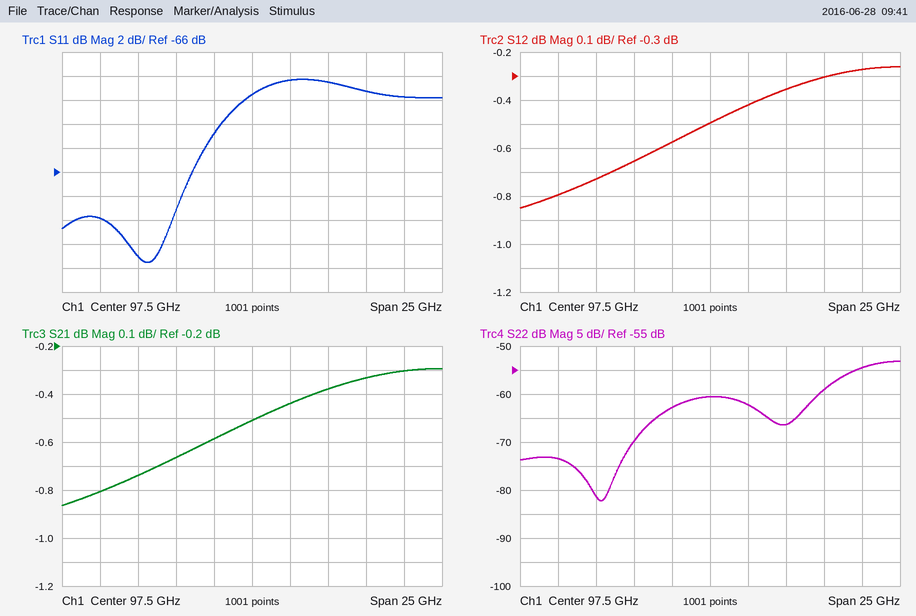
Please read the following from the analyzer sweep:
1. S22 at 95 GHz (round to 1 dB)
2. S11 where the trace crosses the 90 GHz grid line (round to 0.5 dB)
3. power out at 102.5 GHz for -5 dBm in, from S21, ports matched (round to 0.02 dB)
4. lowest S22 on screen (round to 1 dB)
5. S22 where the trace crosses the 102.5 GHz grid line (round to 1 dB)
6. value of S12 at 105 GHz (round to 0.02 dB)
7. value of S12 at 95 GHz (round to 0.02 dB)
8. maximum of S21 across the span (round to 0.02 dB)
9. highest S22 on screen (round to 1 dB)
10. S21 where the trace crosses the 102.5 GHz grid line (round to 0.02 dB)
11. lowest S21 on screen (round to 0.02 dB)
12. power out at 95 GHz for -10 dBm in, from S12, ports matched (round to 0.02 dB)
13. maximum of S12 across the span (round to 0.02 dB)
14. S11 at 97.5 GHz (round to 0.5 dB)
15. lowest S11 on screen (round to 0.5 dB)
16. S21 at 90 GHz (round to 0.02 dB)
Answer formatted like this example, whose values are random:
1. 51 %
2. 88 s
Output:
1. -63 dB
2. -73.0 dB
3. -5.38 dBm
4. -82 dB
5. -66 dB
6. -0.30 dB
7. -0.58 dB
8. -0.30 dB
9. -53 dB
10. -0.38 dB
11. -0.86 dB
12. -10.58 dBm
13. -0.26 dB
14. -59.5 dB
15. -73.5 dB
16. -0.74 dB
